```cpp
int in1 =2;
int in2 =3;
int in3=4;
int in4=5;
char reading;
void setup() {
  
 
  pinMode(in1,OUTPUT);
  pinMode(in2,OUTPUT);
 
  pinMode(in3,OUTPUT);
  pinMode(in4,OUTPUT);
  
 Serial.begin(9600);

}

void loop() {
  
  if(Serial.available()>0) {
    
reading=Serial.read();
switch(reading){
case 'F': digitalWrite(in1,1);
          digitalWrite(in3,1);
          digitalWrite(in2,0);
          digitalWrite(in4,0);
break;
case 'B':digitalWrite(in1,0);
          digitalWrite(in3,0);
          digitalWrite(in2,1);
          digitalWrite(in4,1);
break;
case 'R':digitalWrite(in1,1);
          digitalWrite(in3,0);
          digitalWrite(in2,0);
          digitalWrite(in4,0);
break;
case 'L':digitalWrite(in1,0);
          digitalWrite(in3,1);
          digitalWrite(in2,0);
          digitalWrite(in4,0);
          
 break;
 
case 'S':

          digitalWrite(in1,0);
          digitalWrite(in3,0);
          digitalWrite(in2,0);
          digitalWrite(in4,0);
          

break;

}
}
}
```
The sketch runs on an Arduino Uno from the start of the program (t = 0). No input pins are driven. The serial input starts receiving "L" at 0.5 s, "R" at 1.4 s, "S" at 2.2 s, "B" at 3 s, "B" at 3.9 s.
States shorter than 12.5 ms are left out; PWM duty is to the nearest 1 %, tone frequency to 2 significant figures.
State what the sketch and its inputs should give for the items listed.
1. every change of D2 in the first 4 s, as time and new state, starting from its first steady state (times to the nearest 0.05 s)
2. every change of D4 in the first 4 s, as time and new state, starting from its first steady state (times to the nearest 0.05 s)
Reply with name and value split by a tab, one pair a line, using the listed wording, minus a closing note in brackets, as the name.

every change of D2 in the first 4 s, as time and new state, starting from its first steady state	0 s low; 1.4 s high; 2.2 s low
every change of D4 in the first 4 s, as time and new state, starting from its first steady state	0 s low; 0.5 s high; 1.4 s low
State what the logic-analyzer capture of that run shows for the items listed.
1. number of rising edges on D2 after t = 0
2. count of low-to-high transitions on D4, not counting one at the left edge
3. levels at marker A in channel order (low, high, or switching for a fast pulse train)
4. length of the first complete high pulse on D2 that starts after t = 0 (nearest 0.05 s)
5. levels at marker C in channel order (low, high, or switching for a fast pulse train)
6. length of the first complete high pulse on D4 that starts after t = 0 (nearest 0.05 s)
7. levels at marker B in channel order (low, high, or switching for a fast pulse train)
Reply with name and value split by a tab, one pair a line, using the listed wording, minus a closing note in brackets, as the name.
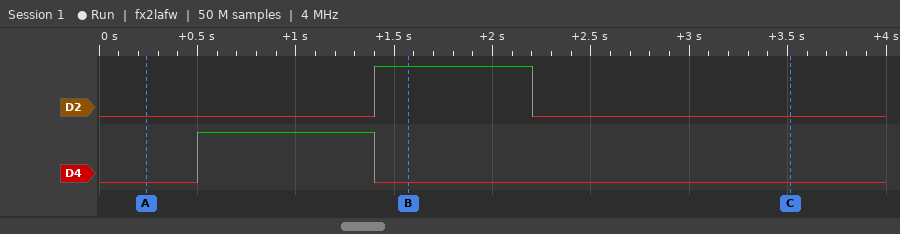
number of rising edges on D2 after t = 0	1
count of low-to-high transitions on D4, not counting one at the left edge	1
levels at marker A in channel order	D2 low, D4 low
length of the first complete high pulse on D2 that starts after t = 0	0.80 s
levels at marker C in channel order	D2 low, D4 low
length of the first complete high pulse on D4 that starts after t = 0	0.90 s
levels at marker B in channel order	D2 high, D4 low
